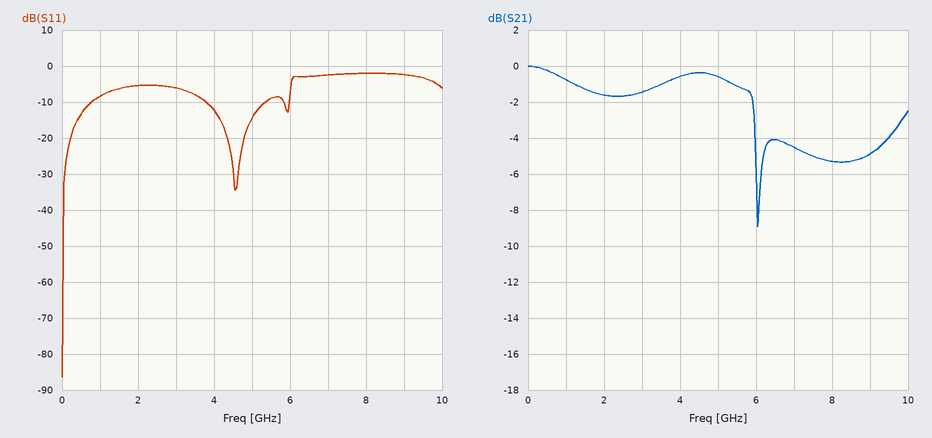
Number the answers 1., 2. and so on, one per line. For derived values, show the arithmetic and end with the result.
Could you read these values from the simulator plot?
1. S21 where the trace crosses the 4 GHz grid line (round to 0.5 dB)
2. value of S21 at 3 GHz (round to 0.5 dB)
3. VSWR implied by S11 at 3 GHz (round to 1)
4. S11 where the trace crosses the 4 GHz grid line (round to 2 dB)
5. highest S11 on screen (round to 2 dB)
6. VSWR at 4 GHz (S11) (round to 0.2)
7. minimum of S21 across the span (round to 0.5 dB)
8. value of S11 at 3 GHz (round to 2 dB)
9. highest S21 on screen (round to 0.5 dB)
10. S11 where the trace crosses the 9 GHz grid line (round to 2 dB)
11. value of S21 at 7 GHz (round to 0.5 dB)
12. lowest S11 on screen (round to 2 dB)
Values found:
1. -0.5 dB
2. -1.5 dB
3. |Γ| = 10^(-6/20) = 0.5012; VSWR = (1 + 0.5012)/(1 − 0.5012) ≈ 3
4. -12 dB
5. -2 dB
6. |Γ| = 10^(-12/20) = 0.2512; VSWR = (1 + 0.2512)/(1 − 0.2512) ≈ 1.67, so 1.6 to the nearest 0.2
7. -9.0 dB
8. -6 dB
9. 0.0 dB
10. -2 dB
11. -4.5 dB
12. -86 dB
